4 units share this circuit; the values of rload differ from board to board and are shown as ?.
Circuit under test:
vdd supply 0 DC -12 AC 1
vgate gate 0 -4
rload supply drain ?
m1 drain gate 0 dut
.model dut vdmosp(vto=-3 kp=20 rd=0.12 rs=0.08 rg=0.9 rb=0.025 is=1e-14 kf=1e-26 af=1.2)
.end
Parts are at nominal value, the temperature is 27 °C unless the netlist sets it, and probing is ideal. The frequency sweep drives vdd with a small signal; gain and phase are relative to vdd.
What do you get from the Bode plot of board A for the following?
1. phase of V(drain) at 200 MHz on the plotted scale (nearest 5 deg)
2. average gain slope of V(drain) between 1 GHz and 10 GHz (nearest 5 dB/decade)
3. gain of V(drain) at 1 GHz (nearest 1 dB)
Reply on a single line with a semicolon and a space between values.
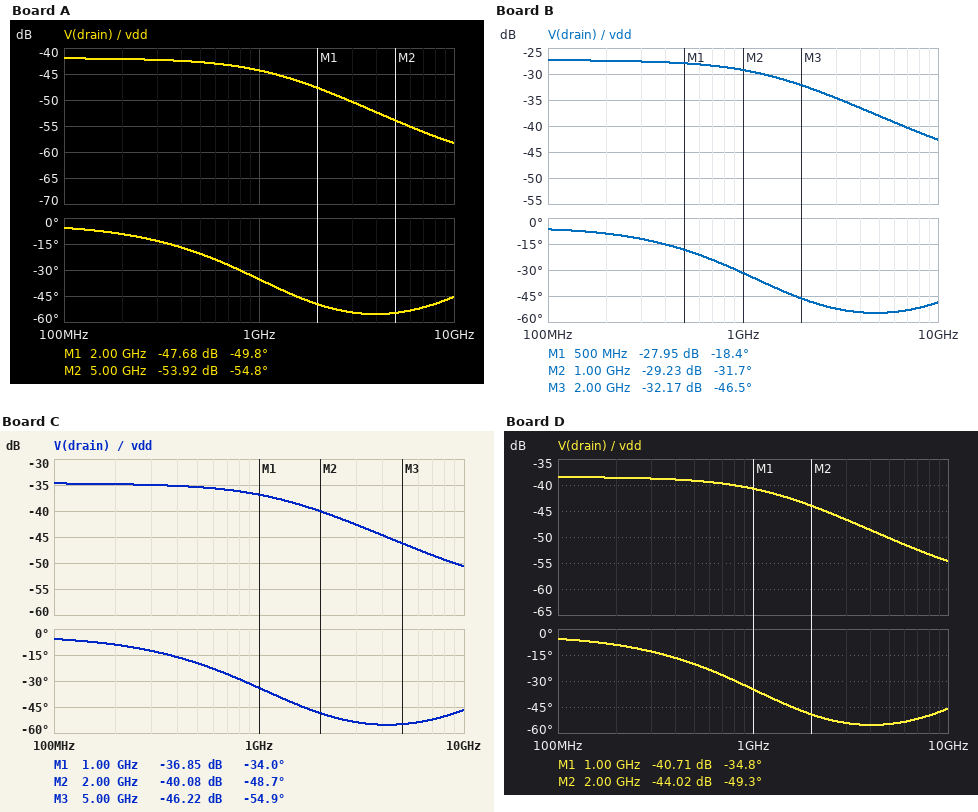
-10 deg; -15 dB/decade; -44 dB
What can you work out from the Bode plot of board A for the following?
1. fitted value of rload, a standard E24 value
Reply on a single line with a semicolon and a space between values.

30 Ω
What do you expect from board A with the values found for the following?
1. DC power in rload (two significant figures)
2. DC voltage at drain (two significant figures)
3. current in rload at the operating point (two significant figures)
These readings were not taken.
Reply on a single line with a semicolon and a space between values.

4.7 W; -100 mV; 400 mA
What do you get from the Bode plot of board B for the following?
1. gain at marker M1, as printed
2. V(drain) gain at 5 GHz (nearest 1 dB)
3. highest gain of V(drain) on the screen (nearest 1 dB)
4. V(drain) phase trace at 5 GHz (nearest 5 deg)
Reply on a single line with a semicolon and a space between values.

-27.95 dB; -38 dB; -27 dB; -55 deg
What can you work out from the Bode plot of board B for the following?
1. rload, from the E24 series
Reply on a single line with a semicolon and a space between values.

5.6 Ω
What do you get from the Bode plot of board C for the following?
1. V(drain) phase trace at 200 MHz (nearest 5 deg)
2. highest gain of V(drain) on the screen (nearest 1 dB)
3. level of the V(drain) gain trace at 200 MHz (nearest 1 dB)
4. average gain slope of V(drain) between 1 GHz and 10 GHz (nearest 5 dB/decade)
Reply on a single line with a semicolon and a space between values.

-10 deg; -35 dB; -35 dB; -15 dB/decade
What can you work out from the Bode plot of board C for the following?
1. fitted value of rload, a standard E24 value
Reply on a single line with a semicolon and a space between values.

13 Ω
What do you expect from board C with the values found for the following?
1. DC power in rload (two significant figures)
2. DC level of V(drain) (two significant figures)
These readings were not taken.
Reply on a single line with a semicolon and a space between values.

11 W; -230 mV
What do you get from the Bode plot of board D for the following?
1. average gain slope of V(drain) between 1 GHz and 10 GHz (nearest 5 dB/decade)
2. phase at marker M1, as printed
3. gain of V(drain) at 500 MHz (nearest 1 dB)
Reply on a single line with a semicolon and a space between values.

-15 dB/decade; -34.8 deg; -39 dB
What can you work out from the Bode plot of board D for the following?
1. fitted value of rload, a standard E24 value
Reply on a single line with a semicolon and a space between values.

20 Ω
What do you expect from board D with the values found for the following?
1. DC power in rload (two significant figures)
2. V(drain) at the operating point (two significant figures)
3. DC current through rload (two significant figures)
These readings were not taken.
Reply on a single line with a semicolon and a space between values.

7.0 W; -150 mV; 590 mA
